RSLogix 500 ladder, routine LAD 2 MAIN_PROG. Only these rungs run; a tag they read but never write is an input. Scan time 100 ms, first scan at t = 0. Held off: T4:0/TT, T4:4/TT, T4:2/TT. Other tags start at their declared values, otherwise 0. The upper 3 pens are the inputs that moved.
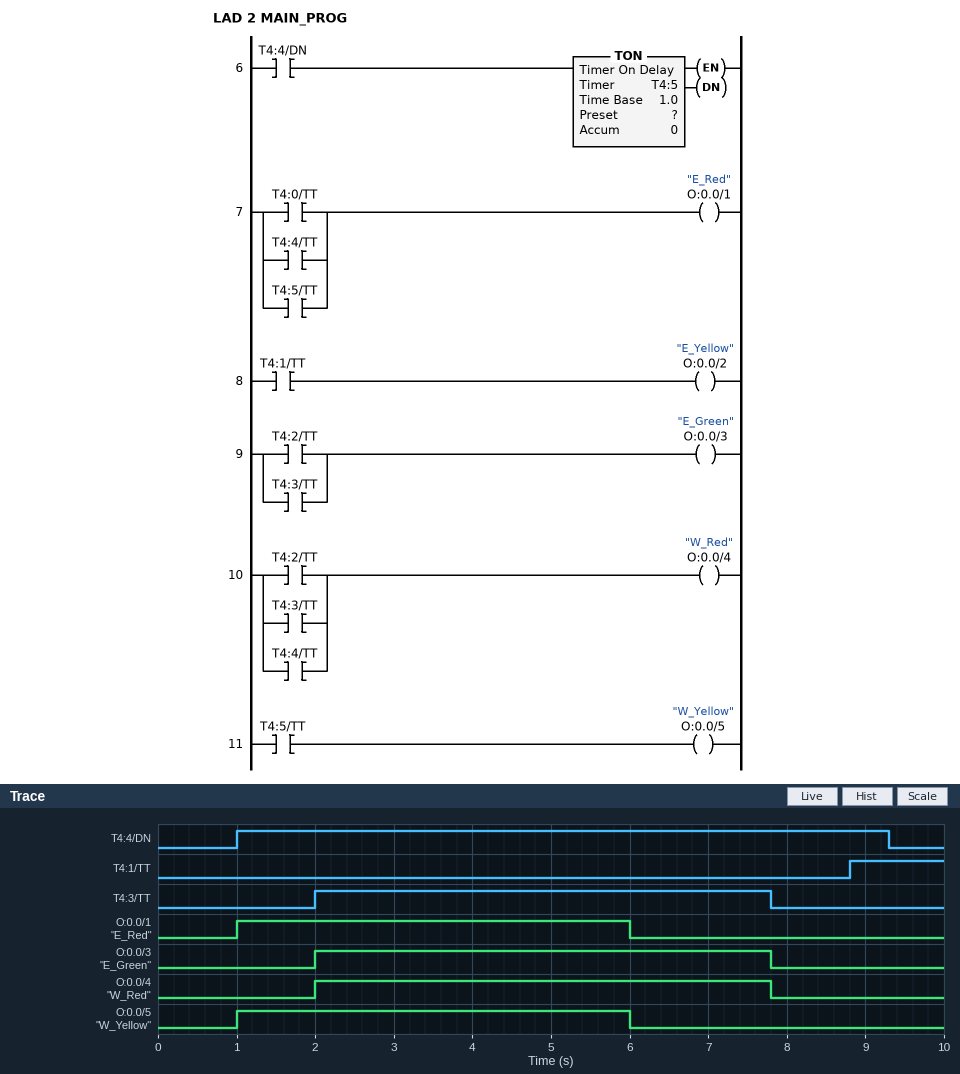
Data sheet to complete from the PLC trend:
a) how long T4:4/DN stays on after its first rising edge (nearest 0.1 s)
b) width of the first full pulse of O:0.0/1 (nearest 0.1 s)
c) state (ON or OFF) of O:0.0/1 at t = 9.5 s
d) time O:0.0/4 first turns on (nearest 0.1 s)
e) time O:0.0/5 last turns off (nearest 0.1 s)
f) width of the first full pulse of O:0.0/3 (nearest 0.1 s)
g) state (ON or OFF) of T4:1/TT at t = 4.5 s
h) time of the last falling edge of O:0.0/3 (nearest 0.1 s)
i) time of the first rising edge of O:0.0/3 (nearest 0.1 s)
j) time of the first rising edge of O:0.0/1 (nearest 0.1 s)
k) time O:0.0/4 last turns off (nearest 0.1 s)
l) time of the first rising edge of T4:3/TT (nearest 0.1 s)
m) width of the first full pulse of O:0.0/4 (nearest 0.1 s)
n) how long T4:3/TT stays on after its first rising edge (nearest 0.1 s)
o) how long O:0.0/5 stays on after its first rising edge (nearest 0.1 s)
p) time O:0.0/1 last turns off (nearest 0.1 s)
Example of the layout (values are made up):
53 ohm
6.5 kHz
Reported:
8.3 s
5.0 s
OFF
2.0 s
6.0 s
5.8 s
OFF
7.8 s
2.0 s
1.0 s
7.8 s
2.0 s
5.8 s
5.8 s
5.0 s
6.0 s
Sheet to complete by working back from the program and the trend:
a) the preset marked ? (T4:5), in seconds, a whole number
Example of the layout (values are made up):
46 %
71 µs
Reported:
5 s
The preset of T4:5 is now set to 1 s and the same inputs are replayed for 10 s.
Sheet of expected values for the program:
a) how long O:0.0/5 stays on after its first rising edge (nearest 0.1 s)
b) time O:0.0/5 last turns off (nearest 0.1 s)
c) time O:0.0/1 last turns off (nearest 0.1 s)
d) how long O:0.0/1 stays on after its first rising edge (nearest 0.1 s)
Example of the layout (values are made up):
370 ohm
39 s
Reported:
1.0 s
2.0 s
2.0 s
1.0 s
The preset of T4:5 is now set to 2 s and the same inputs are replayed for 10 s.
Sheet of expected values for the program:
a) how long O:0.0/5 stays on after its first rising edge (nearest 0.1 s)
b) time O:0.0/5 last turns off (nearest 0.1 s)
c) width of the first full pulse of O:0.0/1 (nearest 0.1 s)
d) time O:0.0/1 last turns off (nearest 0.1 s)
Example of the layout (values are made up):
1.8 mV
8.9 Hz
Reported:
2.0 s
3.0 s
2.0 s
3.0 s
